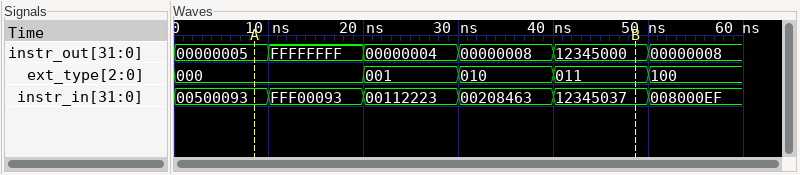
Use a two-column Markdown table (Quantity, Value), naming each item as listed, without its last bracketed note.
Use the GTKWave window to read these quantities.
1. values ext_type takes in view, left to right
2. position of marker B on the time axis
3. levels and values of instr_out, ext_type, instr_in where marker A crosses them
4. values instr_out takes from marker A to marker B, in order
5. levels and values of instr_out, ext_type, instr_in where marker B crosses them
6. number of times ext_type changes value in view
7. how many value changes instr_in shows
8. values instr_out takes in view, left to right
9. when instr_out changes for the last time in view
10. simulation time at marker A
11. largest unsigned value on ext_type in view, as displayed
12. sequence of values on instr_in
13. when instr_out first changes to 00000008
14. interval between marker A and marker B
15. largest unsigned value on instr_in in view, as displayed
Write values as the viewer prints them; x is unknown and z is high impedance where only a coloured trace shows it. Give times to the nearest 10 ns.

| Quantity | Value |
|---|---|
| values ext_type takes in view, left to right | 000, 001, 010, 011, 100 |
| position of marker B on the time axis | 50 ns |
| levels and values of instr_out, ext_type, instr_in where marker A crosses them | instr_out=00000005, ext_type=000, instr_in=00500093 |
| values instr_out takes from marker A to marker B, in order | 00000005, FFFFFFFF, 00000004, 00000008, 12345000 |
| levels and values of instr_out, ext_type, instr_in where marker B crosses them | instr_out=12345000, ext_type=011, instr_in=12345037 |
| number of times ext_type changes value in view | 4 |
| how many value changes instr_in shows | 5 |
| values instr_out takes in view, left to right | 00000005, FFFFFFFF, 00000004, 00000008, 12345000, 00000008 |
| when instr_out changes for the last time in view | 50 ns |
| simulation time at marker A | 10 ns |
| largest unsigned value on ext_type in view, as displayed | 100 |
| sequence of values on instr_in | 00500093, FFF00093, 00112223, 00208463, 12345037, 008000EF |
| when instr_out first changes to 00000008 | 30 ns |
| interval between marker A and marker B | 40 ns |
| largest unsigned value on instr_in in view, as displayed | FFF00093 |
